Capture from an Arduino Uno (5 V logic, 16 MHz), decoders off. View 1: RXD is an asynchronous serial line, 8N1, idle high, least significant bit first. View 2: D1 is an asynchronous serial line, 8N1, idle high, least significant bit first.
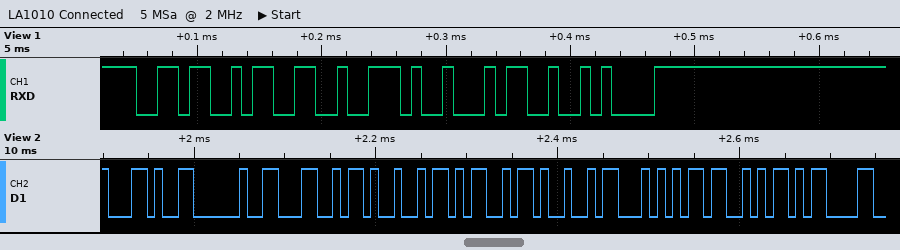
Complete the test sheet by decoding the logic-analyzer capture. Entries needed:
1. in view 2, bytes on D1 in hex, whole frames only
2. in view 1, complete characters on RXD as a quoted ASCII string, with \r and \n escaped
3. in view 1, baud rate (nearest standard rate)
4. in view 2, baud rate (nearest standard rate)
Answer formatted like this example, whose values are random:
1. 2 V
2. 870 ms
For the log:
1. 2C 20 4C 49 4D 49 54 53 0D
2. "63.4\n"
3. 115200 baud
4. 115200 baud
